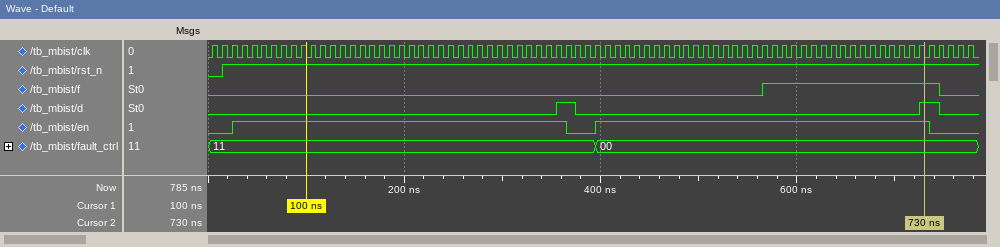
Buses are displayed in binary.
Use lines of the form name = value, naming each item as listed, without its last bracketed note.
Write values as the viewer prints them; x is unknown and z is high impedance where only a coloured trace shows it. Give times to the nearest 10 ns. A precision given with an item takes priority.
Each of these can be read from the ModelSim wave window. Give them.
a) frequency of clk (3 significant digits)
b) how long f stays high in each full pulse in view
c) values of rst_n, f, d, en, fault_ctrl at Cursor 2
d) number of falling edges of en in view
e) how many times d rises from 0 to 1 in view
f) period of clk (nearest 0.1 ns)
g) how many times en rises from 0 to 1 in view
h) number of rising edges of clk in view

frequency of clk = 100 MHz
how long f stays high in each full pulse in view = 180 ns
values of rst_n, f, d, en, fault_ctrl at Cursor 2 = rst_n=1, f=1, d=1, en=1, fault_ctrl=00
number of falling edges of en in view = 2
how many times d rises from 0 to 1 in view = 2
period of clk = 10 ns
how many times en rises from 0 to 1 in view = 2
number of rising edges of clk in view = 78
